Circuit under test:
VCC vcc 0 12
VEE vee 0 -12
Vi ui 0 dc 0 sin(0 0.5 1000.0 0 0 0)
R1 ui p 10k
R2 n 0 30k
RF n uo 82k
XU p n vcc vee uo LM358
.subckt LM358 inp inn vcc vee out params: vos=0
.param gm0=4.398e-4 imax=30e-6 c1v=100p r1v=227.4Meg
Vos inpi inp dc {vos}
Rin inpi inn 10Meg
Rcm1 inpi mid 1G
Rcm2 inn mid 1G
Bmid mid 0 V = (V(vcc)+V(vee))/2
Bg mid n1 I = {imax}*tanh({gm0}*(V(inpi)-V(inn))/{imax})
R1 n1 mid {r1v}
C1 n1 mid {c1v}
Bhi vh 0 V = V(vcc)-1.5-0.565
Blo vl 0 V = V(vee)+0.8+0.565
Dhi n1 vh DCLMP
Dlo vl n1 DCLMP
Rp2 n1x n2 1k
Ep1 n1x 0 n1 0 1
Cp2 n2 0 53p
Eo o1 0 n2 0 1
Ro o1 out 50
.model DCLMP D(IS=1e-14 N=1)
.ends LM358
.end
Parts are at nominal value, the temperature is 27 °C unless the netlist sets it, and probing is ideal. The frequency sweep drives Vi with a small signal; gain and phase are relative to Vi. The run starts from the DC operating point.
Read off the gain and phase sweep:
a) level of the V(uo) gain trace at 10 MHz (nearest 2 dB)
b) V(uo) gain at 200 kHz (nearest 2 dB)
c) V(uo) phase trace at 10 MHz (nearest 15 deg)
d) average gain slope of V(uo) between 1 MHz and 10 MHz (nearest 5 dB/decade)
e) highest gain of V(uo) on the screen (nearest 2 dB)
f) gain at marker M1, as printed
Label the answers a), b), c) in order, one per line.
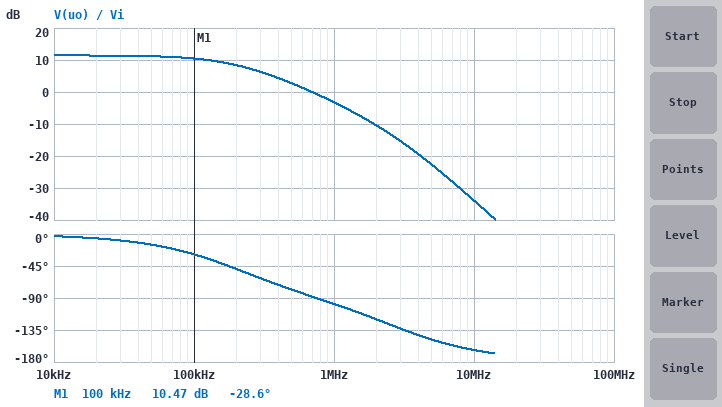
a) -34 dB
b) 8 dB
c) -165 deg
d) -30 dB/decade
e) 12 dB
f) 10.47 dB
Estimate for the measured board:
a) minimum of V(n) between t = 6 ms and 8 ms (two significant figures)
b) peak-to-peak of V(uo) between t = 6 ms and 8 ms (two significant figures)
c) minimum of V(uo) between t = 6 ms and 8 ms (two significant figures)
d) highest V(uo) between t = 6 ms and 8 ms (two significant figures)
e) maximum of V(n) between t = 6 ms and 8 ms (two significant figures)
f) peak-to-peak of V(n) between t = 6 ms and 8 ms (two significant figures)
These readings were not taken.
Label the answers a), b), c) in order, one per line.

a) -500 mV
b) 3.7 V
c) -1.9 V
d) 1.9 V
e) 500 mV
f) 1.0 V
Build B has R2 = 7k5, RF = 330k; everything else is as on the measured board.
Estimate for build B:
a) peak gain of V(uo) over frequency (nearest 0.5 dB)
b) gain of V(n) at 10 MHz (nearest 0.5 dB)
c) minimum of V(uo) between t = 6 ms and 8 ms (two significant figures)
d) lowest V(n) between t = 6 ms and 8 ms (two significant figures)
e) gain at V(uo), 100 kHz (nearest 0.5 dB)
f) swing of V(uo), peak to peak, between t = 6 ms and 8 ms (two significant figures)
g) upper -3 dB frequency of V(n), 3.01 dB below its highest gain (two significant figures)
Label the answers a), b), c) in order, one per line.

a) 33.0 dB
b) -69.5 dB
c) -11 V
d) -250 mV
e) 17.0 dB
f) 22 V
g) 16 kHz
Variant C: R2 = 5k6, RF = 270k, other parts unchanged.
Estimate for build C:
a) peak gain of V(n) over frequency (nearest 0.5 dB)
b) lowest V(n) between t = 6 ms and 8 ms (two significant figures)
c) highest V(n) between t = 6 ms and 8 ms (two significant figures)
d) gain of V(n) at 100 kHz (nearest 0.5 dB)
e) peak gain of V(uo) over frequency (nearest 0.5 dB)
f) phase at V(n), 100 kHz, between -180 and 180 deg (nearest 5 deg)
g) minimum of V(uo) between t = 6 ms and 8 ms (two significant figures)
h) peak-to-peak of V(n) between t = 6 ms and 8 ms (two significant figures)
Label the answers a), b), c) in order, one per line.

a) 0 dB
b) -230 mV
c) 210 mV
d) -17.0 dB
e) 34.0 dB
f) -85 deg
g) -11 V
h) 440 mV
